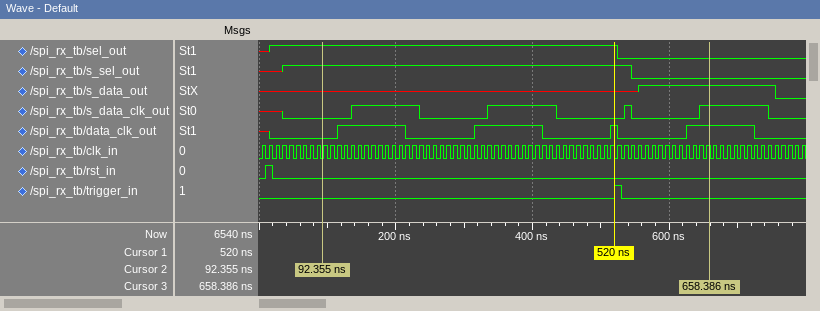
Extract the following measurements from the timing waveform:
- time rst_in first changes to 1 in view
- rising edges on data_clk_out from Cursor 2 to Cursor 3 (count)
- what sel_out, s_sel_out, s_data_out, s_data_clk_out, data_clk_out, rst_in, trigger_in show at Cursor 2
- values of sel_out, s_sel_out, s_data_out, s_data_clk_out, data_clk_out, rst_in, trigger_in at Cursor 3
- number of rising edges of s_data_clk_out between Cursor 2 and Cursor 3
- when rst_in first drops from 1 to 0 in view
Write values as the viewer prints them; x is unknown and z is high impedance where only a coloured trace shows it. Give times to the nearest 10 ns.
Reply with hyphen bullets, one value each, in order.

- 10 ns
- 4
- sel_out=1, s_sel_out=1, s_data_out=x, s_data_clk_out=0, data_clk_out=0, rst_in=0, trigger_in=0
- sel_out=0, s_sel_out=0, s_data_out=1, s_data_clk_out=1, data_clk_out=1, rst_in=0, trigger_in=0
- 4
- 20 ns
